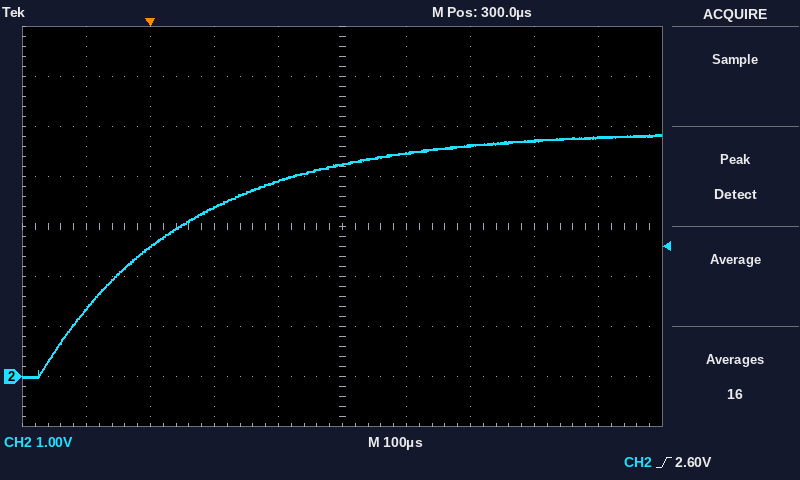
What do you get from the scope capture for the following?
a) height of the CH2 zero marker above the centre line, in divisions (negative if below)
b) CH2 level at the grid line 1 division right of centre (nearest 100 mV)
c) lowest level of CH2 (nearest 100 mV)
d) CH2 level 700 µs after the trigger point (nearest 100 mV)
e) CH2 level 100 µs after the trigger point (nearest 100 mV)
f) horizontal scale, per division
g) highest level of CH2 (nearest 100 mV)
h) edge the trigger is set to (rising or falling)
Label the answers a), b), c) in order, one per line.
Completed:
a) -3.0 div
b) 4.5 V
c) 0.0 V
d) 4.8 V
e) 3.4 V
f) 100 µs
g) 4.8 V
h) rising
